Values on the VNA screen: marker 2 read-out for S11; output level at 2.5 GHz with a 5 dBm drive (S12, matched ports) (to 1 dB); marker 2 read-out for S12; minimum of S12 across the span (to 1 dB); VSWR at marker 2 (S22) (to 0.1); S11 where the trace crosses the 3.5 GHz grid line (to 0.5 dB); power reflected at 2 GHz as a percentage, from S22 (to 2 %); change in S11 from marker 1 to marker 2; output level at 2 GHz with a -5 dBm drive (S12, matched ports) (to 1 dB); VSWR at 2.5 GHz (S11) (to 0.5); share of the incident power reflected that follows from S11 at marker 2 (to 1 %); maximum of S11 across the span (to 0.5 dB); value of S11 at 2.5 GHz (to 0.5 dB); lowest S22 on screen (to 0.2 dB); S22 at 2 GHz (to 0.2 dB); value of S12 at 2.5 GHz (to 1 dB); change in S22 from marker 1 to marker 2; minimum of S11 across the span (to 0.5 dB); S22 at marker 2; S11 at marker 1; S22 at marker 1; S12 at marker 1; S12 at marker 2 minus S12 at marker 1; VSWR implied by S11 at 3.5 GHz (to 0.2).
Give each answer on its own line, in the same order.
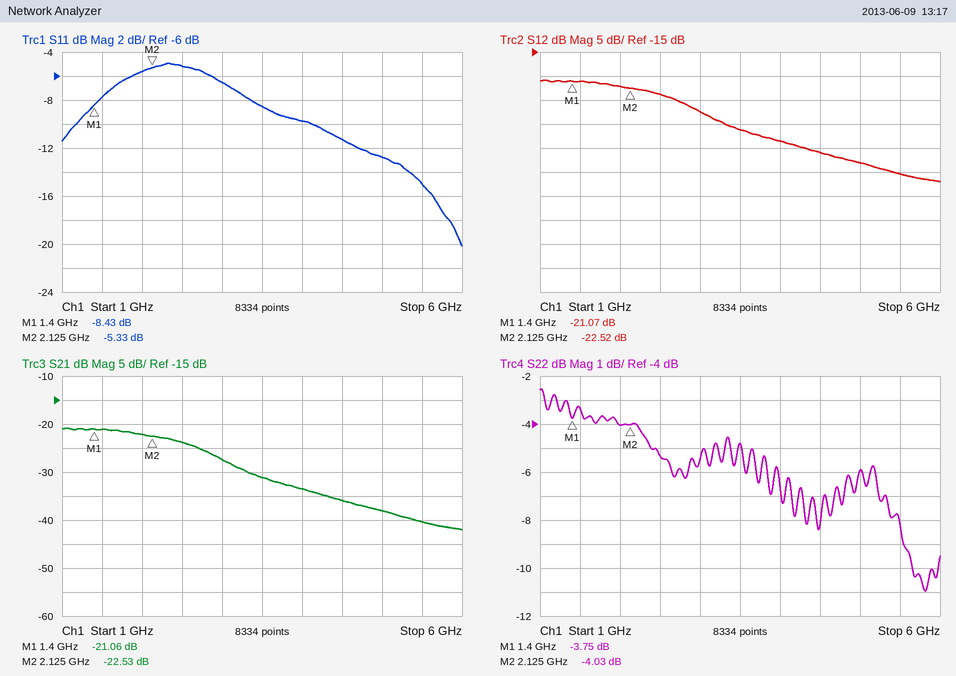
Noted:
-5.33 dB
-19 dBm
-22.52 dB
-42 dB
4.4
-8.5 dB
40 %
3.10 dB
-27 dBm
3.5
29 %
-5.0 dB
-5.0 dB
-11.0 dB
-4.0 dB
-24 dB
-0.28 dB
-20.0 dB
-4.03 dB
-8.43 dB
-3.75 dB
-21.07 dB
-1.45 dB
2.2
